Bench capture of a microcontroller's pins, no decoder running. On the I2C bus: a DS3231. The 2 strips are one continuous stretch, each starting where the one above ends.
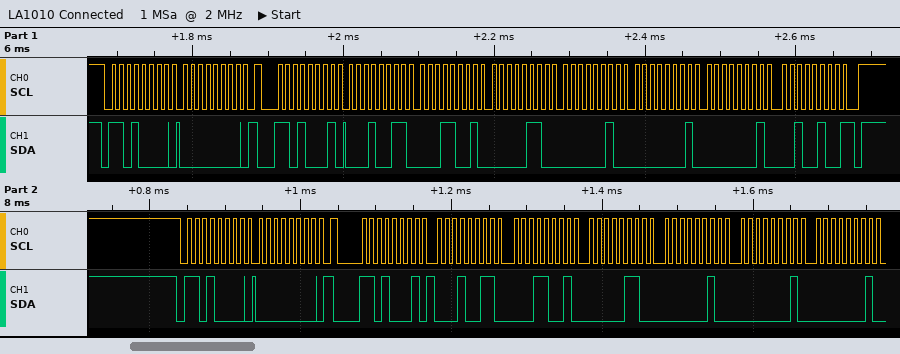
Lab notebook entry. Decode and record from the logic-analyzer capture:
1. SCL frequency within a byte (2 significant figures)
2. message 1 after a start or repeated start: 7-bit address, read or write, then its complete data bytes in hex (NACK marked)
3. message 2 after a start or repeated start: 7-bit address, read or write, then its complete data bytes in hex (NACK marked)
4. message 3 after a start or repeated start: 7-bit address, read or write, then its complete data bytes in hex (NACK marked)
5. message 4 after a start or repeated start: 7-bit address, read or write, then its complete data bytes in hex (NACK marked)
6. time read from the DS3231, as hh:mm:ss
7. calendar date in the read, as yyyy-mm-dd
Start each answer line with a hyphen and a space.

- 100 kHz
- 0x68 write: 00
- 0x68 read: 13 19 06 02 01 01 24 NACK
- 0x68 write: 00
- 0x68 read: 13 19 06 02 01 01
- 06:19:13
- 2024-01-01
